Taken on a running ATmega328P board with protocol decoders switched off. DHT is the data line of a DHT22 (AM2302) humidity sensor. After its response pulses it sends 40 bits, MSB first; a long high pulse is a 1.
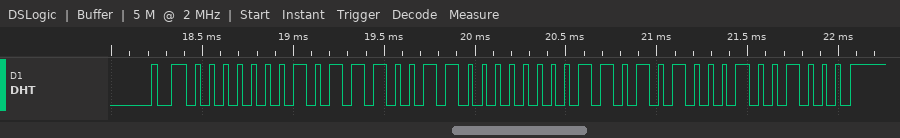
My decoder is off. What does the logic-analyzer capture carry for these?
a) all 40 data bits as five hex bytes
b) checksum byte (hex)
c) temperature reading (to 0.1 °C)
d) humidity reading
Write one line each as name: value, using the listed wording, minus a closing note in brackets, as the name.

all 40 data bits as five hex bytes: 01 73 00 D4 48
checksum byte: 0x48
temperature reading: 21.2 °C
humidity reading: 37.1 %
